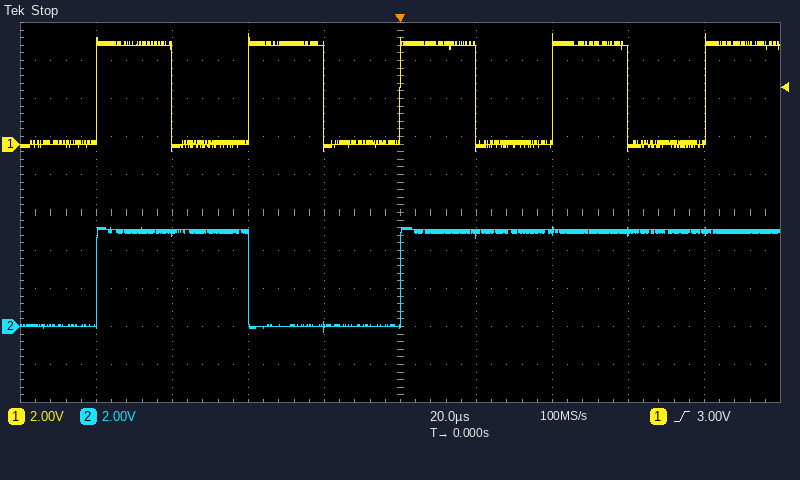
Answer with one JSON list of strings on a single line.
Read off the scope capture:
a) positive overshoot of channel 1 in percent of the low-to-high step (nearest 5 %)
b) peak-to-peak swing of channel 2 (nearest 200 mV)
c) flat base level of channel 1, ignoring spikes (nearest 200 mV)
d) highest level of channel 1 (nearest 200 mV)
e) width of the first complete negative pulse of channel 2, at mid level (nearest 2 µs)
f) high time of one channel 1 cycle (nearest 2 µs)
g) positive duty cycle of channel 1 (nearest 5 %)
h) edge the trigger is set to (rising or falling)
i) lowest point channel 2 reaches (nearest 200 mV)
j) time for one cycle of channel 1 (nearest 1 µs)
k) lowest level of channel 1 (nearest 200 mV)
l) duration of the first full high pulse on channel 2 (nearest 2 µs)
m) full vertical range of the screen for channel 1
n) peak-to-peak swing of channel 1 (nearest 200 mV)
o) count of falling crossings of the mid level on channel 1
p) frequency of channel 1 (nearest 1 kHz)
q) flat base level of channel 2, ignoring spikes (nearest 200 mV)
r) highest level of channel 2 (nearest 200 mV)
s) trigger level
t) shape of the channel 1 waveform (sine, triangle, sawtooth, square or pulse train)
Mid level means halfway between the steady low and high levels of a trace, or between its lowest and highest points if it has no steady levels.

["10 %", "5.6 V", "0.0 V", "5.8 V", "40 µs", "20 µs", "50 %", "rising", "-400 mV", "40 µs", "-400 mV", "40 µs", "20 V", "6.2 V", "4", "25 kHz", "0.0 V", "5.2 V", "3.00 V", "square"]
